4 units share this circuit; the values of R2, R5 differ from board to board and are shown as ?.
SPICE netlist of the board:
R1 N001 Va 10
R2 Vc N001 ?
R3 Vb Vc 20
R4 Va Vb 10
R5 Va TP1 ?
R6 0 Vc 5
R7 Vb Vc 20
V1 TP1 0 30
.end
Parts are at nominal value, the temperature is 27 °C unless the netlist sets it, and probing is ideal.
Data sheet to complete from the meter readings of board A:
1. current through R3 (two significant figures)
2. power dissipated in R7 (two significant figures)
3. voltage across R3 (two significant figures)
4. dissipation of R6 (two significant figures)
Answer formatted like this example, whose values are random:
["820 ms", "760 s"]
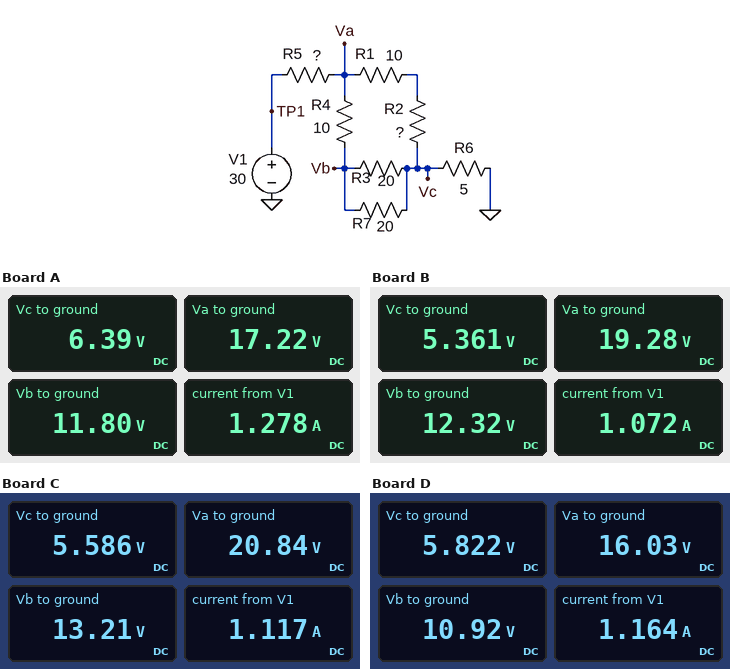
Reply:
["270 mA", "1.5 W", "5.4 V", "8.2 W"]
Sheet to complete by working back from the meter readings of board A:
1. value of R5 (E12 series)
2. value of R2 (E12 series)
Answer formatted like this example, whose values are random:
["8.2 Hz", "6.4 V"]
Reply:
["10 Ω", "4.7 Ω"]
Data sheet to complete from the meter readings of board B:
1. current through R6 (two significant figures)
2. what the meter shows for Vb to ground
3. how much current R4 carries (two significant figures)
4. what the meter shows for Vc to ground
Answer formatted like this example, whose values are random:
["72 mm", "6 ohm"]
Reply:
["1.1 A", "12.32 V", "700 mA", "5.361 V"]
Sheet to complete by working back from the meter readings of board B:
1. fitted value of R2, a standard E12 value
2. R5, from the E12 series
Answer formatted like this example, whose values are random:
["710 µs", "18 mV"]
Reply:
["27 Ω", "10 Ω"]
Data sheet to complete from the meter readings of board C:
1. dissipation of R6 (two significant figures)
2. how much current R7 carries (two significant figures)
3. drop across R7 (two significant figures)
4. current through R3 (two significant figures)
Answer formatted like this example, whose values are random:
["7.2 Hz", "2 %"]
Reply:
["6.2 W", "380 mA", "7.6 V", "380 mA"]
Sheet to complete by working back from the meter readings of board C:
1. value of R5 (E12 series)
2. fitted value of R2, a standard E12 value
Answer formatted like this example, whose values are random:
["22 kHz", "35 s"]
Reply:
["8.2 Ω", "33 Ω"]
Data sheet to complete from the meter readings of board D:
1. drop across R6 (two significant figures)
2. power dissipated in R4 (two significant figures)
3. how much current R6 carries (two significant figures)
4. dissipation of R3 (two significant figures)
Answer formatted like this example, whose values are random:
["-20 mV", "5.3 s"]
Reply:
["5.8 V", "2.6 W", "1.2 A", "1.3 W"]
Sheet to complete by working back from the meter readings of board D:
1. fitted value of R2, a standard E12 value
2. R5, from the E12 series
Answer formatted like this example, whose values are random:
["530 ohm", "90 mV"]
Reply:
["5.6 Ω", "12 Ω"]
